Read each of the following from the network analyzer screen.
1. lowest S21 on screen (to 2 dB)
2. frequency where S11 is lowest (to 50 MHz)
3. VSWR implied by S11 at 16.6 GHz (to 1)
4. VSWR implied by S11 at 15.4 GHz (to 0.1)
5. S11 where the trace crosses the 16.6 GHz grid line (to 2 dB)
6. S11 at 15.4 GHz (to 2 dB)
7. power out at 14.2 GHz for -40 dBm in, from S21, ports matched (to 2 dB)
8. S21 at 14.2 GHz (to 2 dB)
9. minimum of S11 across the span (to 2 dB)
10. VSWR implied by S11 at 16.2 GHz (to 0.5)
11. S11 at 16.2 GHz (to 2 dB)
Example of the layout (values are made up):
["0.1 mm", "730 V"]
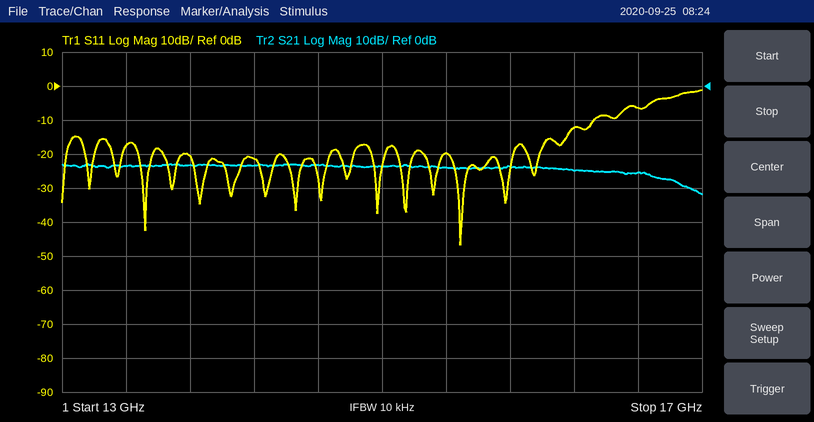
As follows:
["-32 dB", "15.50 GHz", "3", "1.2", "-6 dB", "-20 dB", "-64 dBm", "-24 dB", "-46 dB", "1.5", "-12 dB"]
